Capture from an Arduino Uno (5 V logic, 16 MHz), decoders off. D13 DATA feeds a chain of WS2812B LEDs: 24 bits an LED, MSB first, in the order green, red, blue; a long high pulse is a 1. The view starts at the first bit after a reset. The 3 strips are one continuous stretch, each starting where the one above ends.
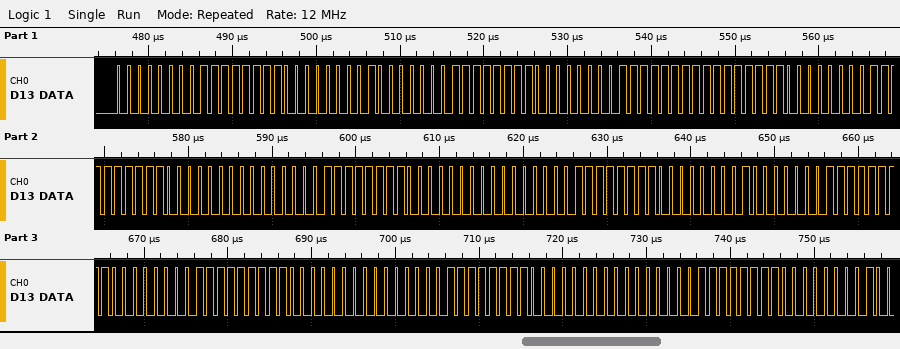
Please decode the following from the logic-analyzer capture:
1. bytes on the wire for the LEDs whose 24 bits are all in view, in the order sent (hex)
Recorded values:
00 FF 00 80 FF 00 FF FF 00 FF 80 00 FF 00 00 FF 00 80 FF 00 FF 80 00 FF 00 00 FF
